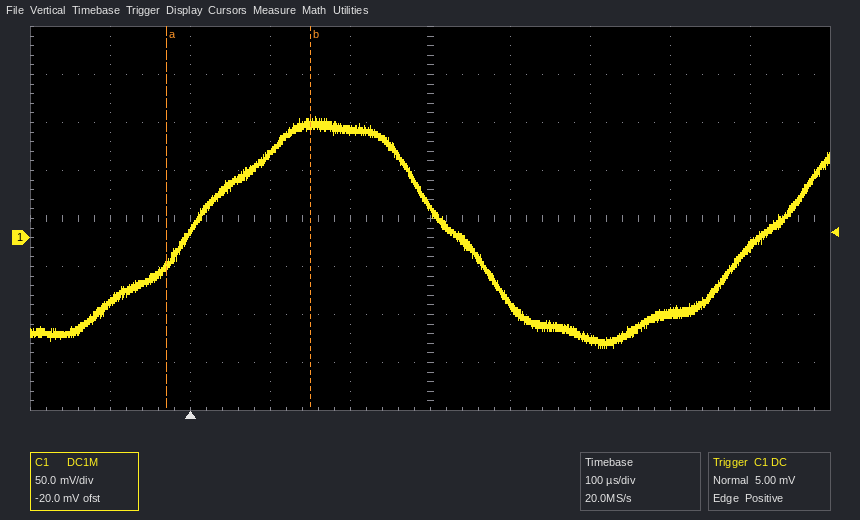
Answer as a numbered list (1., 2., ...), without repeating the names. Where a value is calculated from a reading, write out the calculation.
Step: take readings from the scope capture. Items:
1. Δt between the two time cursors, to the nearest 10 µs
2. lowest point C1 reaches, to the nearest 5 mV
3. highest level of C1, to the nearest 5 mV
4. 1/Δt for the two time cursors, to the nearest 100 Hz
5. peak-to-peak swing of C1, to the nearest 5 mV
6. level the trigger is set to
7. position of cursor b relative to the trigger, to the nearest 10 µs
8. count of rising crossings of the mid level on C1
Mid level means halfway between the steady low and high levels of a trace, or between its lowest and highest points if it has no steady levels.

1. 180 µs
2. -115 mV
3. 125 mV
4. 1 / 180 µs ≈ 5.6 kHz
5. 125 mV − (-115 mV) = 240 mV
6. 5.00 mV
7. +150 µs
8. 2
